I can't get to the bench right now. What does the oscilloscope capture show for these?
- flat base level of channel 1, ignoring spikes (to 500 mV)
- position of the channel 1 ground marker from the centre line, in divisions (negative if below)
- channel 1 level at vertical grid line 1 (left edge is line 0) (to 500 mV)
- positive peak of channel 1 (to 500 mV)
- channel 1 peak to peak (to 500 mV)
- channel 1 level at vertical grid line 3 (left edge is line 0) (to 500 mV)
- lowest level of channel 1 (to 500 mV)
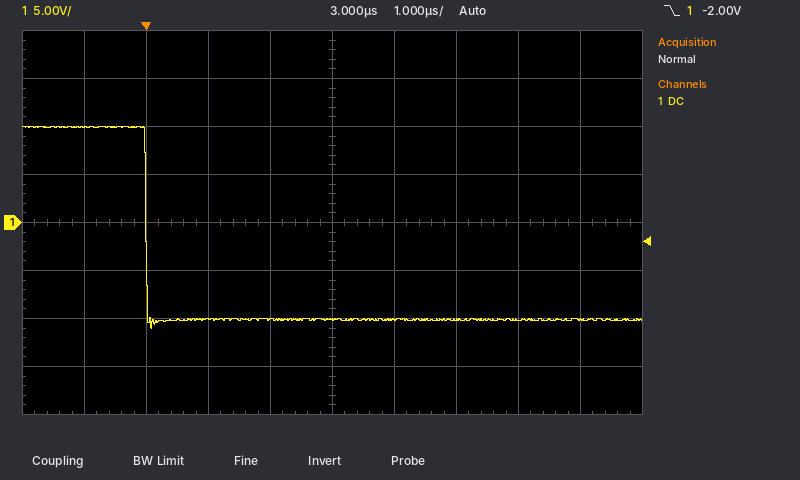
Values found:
-10.0 V
0.0 div
10.0 V
10.0 V
21.0 V
-10.0 V
-11.0 V
